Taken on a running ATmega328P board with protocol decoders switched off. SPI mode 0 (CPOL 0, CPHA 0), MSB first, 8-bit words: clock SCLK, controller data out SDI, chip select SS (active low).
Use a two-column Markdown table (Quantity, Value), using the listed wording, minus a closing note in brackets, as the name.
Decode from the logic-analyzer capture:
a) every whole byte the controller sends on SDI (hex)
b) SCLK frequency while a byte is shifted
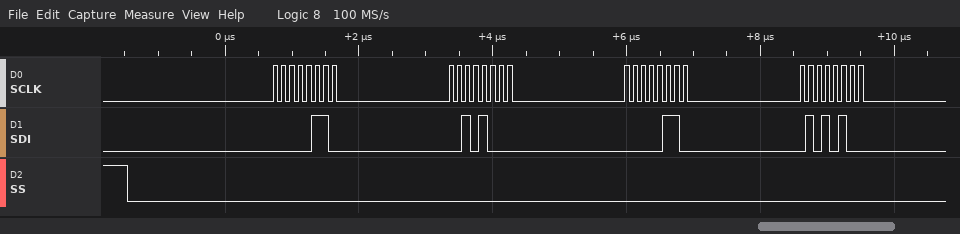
| Quantity | Value |
|---|---|
| every whole byte the controller sends on SDI | 0x06 0x28 0x06 0x54 |
| SCLK frequency while a byte is shifted | 8 MHz |
